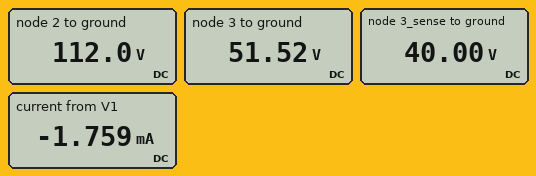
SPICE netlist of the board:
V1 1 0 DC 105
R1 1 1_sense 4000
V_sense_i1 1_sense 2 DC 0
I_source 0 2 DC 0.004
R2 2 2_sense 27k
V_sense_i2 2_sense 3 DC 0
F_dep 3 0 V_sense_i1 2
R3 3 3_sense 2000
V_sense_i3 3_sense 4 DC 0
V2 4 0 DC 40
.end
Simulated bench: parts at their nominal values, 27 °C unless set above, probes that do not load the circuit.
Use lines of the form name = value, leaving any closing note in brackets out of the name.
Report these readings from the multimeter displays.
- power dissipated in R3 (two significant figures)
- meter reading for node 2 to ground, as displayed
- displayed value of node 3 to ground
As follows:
power dissipated in R3 = 66 mW
meter reading for node 2 to ground, as displayed = 112.0 V
displayed value of node 3 to ground = 51.52 V
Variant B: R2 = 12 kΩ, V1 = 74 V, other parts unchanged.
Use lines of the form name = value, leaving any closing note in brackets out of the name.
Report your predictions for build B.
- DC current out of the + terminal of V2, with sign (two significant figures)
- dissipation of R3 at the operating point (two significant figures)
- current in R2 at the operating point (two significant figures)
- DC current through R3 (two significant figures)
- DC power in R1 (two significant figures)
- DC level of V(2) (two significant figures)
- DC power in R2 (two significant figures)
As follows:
DC current out of the + terminal of V2, with sign = -5.6 mA
dissipation of R3 at the operating point = 62 mW
current in R2 at the operating point = 2.4 mA
DC current through R3 = 5.6 mA
DC power in R1 = 9.9 mW
DC level of V(2) = 80 V
DC power in R2 = 71 mW
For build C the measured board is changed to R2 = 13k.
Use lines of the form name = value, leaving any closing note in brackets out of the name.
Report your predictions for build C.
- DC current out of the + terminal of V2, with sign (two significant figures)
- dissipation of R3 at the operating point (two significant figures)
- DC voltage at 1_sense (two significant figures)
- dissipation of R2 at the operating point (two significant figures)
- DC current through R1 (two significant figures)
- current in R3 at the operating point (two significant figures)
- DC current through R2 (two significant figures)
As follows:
DC current out of the + terminal of V2, with sign = -3.7 mA
dissipation of R3 at the operating point = 27 mW
DC voltage at 1_sense = 100 V
dissipation of R2 at the operating point = 240 mW
DC current through R1 = 330 µA
current in R3 at the operating point = 3.7 mA
DC current through R2 = 4.3 mA
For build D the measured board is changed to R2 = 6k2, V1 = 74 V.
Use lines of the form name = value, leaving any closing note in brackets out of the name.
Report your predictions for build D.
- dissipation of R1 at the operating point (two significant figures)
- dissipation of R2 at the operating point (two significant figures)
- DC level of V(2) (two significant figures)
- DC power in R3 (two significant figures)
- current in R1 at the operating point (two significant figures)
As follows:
dissipation of R1 at the operating point = 86 µW
dissipation of R2 at the operating point = 110 mW
DC level of V(2) = 73 V
DC power in R3 = 30 mW
current in R1 at the operating point = 150 µA
